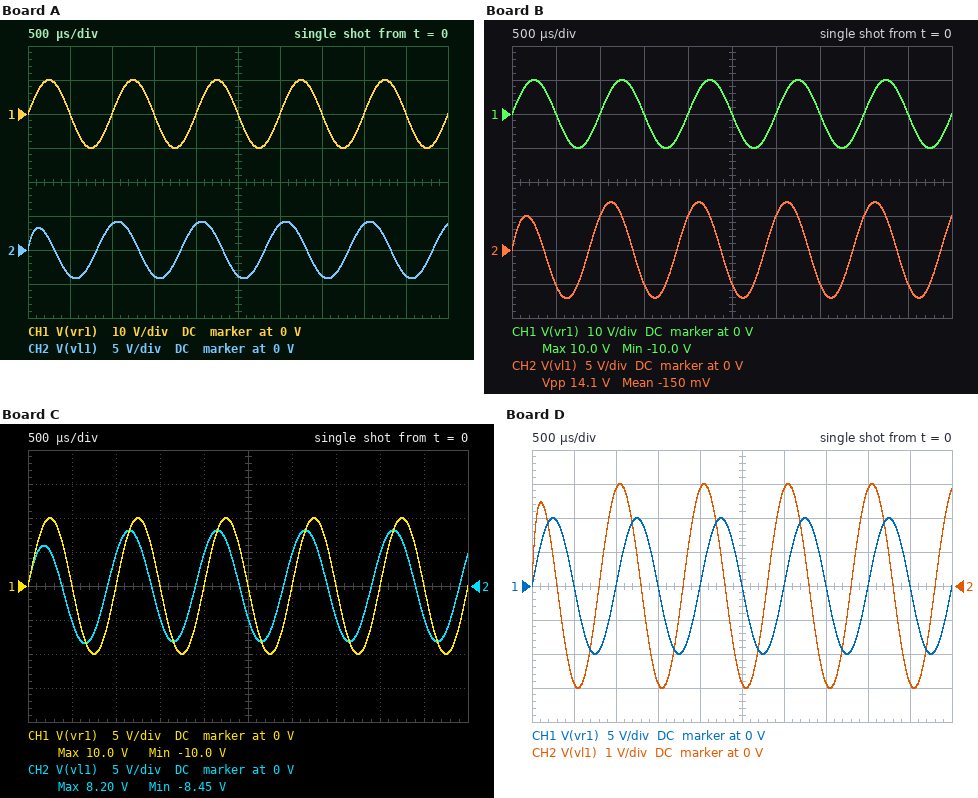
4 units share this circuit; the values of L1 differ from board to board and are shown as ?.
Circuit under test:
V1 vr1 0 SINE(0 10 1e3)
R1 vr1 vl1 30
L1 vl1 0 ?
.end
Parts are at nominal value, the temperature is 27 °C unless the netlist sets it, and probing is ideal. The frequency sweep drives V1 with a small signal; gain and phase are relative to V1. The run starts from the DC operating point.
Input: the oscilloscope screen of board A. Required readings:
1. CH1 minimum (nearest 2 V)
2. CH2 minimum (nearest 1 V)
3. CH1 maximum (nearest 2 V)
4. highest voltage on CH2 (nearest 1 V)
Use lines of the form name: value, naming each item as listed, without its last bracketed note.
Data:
CH1 minimum: -10 V
CH2 minimum: -4 V
CH1 maximum: 10 V
highest voltage on CH2: 4 V
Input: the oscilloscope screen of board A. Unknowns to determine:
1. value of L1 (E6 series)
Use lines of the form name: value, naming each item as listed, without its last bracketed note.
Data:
value of L1: 2.2 mH
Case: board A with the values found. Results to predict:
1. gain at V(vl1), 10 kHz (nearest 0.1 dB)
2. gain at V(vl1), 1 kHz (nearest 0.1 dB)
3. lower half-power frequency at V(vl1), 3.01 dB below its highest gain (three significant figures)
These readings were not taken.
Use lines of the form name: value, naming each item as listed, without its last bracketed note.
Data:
gain at V(vl1), 10 kHz: -0.2 dB
gain at V(vl1), 1 kHz: -7.6 dB
lower half-power frequency at V(vl1), 3.01 dB below its highest gain: 2.17 kHz
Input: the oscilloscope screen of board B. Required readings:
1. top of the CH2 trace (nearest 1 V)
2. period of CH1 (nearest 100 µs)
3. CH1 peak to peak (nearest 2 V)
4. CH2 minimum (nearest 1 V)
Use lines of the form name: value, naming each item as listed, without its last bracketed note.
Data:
top of the CH2 trace: 7 V
period of CH1: 1.0 ms
CH1 peak to peak: 20 V
CH2 minimum: -7 V
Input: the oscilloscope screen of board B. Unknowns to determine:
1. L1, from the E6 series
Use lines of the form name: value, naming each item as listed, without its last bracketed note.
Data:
L1, from the E6 series: 4.7 mH
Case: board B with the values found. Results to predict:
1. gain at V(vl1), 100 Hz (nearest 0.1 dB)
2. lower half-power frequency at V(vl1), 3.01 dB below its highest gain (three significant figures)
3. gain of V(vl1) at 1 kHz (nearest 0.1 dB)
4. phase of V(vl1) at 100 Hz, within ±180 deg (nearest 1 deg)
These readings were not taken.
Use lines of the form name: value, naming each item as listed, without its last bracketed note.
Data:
gain at V(vl1), 100 Hz: -20.2 dB
lower half-power frequency at V(vl1), 3.01 dB below its highest gain: 1.02 kHz
gain of V(vl1) at 1 kHz: -3.1 dB
phase of V(vl1) at 100 Hz, within ±180 deg: 84 deg
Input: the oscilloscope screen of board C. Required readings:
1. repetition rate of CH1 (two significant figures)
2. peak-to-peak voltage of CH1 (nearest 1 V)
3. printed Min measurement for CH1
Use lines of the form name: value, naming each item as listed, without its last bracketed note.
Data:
repetition rate of CH1: 1.0 kHz
peak-to-peak voltage of CH1: 20 V
printed Min measurement for CH1: -10.0 V
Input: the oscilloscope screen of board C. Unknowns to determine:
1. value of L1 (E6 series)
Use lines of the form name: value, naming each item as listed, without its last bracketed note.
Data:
value of L1: 6.8 mH
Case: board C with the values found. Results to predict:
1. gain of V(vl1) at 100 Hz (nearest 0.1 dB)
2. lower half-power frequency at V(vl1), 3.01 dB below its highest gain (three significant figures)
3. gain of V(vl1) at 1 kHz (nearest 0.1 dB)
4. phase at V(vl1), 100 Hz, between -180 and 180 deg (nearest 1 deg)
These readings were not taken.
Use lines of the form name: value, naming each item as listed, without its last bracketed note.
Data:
gain of V(vl1) at 100 Hz: -17.0 dB
lower half-power frequency at V(vl1), 3.01 dB below its highest gain: 702 Hz
gain of V(vl1) at 1 kHz: -1.7 dB
phase at V(vl1), 100 Hz, between -180 and 180 deg: 82 deg
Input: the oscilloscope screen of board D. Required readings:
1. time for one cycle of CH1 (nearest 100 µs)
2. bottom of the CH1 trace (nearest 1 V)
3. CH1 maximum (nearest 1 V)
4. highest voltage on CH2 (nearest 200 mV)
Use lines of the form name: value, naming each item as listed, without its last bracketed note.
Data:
time for one cycle of CH1: 1.0 ms
bottom of the CH1 trace: -10 V
CH1 maximum: 10 V
highest voltage on CH2: 3.0 V
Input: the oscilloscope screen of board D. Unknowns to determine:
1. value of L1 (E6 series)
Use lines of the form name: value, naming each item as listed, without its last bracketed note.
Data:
value of L1: 1.5 mH
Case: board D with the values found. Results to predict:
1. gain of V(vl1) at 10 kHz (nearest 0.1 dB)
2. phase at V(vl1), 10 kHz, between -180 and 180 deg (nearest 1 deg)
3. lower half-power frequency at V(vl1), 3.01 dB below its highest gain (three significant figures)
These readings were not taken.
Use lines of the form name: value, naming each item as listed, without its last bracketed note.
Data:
gain of V(vl1) at 10 kHz: -0.4 dB
phase at V(vl1), 10 kHz, between -180 and 180 deg: 18 deg
lower half-power frequency at V(vl1), 3.01 dB below its highest gain: 3.18 kHz
